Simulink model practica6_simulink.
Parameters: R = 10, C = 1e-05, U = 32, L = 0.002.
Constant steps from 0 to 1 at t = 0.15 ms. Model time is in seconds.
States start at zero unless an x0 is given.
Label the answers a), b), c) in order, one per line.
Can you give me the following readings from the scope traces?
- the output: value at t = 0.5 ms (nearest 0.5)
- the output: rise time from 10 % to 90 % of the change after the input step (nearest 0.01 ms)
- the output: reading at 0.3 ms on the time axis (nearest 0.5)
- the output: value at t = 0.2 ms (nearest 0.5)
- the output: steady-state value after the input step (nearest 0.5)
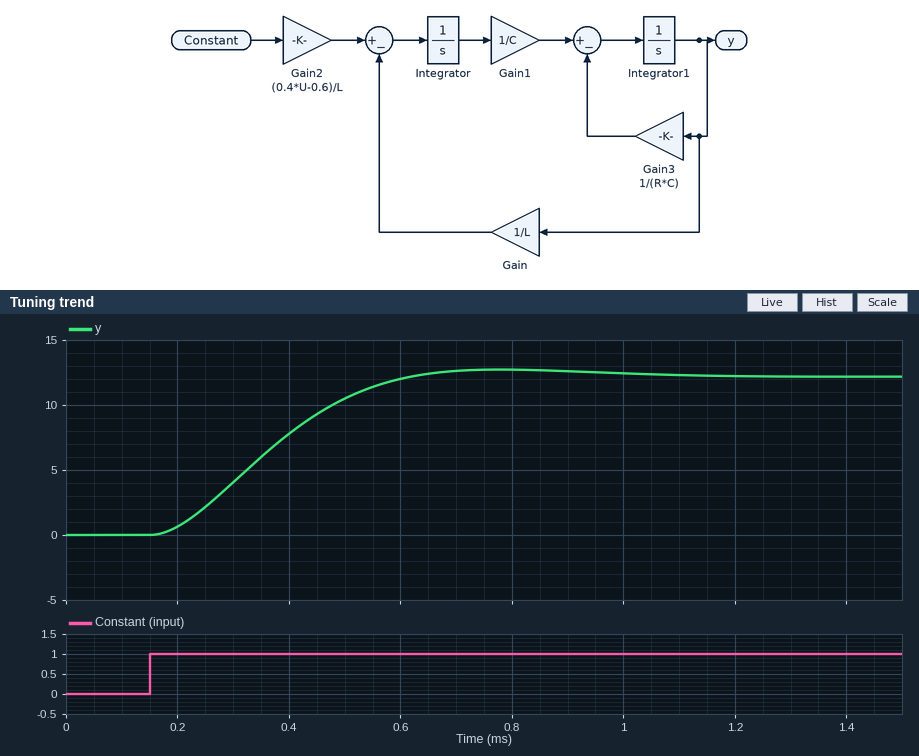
a) 10.5
b) 0.30 ms
c) 4.0
d) 0.5
e) 12.0
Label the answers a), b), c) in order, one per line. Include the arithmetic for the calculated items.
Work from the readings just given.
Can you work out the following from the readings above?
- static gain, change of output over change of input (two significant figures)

a) (12 - 0) / (1 - 0) = 12
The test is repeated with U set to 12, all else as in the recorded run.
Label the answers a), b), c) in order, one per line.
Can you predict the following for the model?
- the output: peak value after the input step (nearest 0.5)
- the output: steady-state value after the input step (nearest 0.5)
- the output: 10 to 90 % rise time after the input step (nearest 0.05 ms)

a) 4.5
b) 4.0
c) 0.30 ms
